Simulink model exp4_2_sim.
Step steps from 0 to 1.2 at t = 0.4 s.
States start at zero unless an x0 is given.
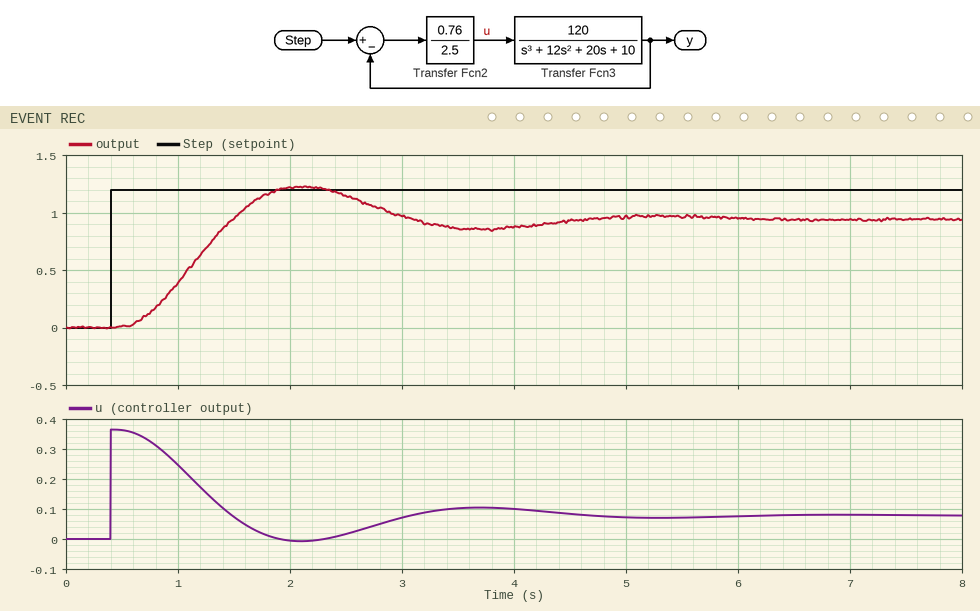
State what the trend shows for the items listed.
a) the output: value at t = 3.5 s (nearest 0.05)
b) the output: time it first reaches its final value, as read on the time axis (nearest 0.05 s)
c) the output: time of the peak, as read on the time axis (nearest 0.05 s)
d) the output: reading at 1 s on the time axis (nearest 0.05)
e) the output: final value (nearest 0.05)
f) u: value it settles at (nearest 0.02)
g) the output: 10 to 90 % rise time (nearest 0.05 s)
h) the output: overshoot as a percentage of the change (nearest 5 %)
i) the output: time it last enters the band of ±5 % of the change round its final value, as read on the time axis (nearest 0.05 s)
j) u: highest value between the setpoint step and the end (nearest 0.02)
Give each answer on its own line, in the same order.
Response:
0.85
1.50 s
2.10 s
0.40
0.95
0.08
0.70 s
30 %
4.25 s
0.36
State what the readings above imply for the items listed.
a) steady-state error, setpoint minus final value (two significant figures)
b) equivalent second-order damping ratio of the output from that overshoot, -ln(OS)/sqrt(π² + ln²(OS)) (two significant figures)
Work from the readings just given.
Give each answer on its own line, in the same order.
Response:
0.25
0.36
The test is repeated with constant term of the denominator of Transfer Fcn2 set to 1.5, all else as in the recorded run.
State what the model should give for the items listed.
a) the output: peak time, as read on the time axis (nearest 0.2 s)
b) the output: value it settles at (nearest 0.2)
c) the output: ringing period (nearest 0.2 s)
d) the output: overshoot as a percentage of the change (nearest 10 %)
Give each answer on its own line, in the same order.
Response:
1.8 s
1.0
2.6 s
40 %
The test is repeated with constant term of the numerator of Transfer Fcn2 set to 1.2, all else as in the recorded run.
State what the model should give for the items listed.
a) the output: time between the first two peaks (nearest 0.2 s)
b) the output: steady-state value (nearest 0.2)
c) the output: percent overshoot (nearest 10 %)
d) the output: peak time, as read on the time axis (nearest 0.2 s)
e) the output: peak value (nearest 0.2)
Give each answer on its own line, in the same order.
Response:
2.6 s
1.0
40 %
1.8 s
1.4
